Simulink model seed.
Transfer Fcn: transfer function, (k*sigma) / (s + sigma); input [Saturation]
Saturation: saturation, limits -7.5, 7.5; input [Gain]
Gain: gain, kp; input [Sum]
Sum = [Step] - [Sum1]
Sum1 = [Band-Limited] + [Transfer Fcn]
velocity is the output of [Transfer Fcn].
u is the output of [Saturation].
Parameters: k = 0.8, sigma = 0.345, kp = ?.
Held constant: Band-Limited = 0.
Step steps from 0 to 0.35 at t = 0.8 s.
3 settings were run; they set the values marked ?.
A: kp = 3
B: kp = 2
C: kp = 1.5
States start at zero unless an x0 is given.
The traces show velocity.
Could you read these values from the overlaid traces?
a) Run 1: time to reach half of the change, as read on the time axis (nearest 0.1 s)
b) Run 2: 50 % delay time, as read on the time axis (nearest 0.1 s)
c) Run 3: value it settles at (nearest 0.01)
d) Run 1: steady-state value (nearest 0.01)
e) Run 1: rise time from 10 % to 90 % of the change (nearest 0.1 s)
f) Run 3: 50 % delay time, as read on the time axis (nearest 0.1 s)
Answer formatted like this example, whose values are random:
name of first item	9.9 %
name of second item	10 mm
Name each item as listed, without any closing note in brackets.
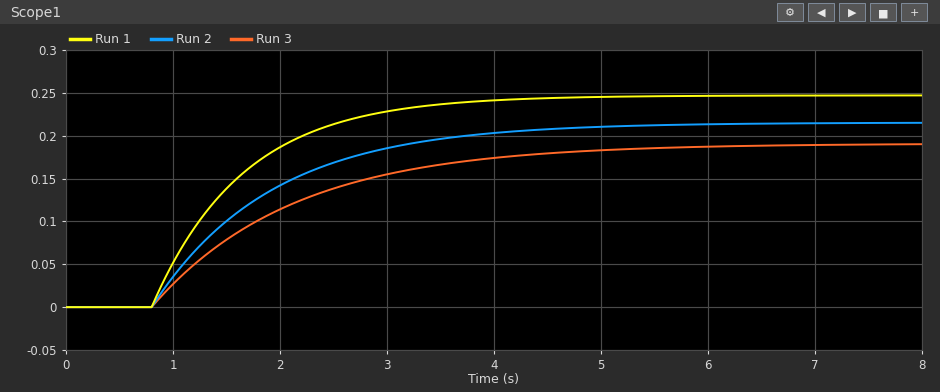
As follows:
Run 1: time to reach half of the change, as read on the time axis	1.4 s
Run 2: 50 % delay time, as read on the time axis	1.6 s
Run 3: value it settles at	0.19
Run 1: steady-state value	0.25
Run 1: rise time from 10 % to 90 % of the change	1.9 s
Run 3: 50 % delay time, as read on the time axis	1.7 s
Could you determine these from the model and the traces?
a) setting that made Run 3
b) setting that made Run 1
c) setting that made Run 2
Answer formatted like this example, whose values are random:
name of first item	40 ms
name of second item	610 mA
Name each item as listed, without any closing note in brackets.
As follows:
setting that made Run 3	C
setting that made Run 1	A
setting that made Run 2	B
